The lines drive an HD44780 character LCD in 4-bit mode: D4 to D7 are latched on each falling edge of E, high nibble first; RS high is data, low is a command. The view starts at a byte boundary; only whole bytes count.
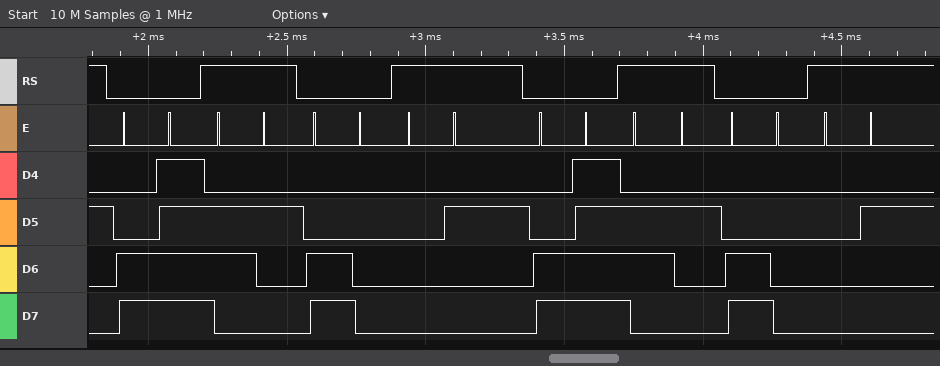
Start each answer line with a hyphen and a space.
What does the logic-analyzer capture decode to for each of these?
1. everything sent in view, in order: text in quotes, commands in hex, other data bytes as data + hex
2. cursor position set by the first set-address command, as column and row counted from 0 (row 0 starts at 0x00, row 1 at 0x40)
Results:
- 0xCF "b" 0xC0 data 02 0xCF "b" 0xC0 data 02
- column 15, row 1
